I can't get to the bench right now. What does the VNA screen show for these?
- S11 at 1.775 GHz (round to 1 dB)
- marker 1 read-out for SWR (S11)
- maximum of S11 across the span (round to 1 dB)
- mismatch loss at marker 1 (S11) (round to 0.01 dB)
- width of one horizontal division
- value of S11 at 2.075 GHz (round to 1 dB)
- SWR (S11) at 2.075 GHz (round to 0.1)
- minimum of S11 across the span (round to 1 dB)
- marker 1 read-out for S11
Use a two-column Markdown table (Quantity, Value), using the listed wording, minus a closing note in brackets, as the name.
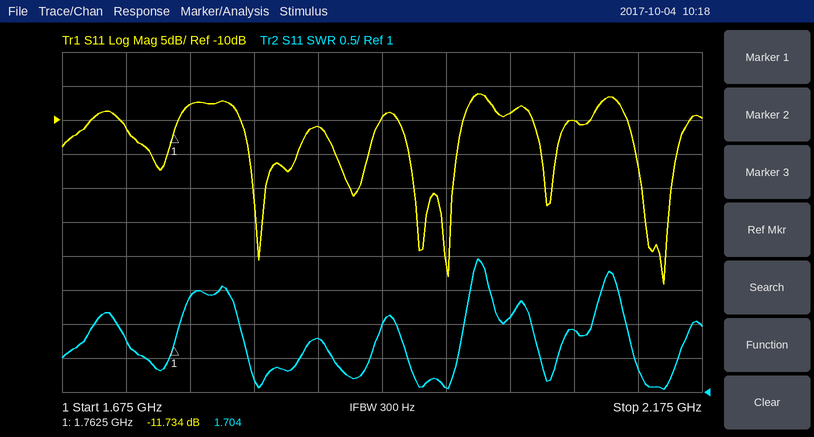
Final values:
| Quantity | Value |
|---|---|
| S11 at 1.775 GHz | -8 dB |
| marker 1 read-out for SWR | 1.704 |
| maximum of S11 across the span | -6 dB |
| mismatch loss at marker 1 (S11) | 0.30 dB |
| width of one horizontal division | 50 MHz |
| value of S11 at 2.075 GHz | -10 dB |
| SWR (S11) at 2.075 GHz | 1.9 |
| minimum of S11 across the span | -34 dB |
| marker 1 read-out for S11 | -11.734 dB |
